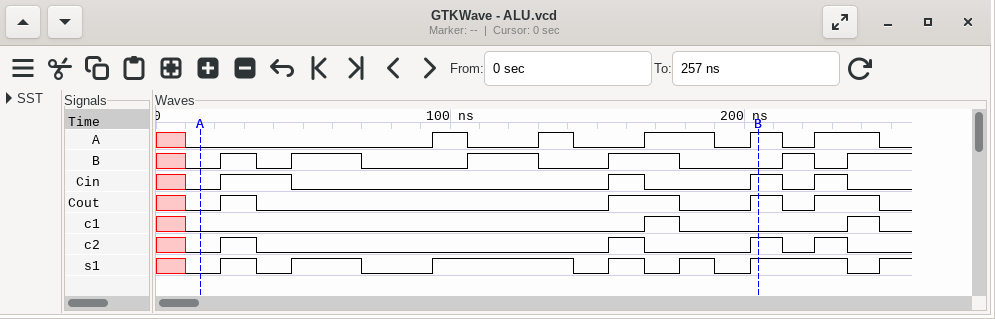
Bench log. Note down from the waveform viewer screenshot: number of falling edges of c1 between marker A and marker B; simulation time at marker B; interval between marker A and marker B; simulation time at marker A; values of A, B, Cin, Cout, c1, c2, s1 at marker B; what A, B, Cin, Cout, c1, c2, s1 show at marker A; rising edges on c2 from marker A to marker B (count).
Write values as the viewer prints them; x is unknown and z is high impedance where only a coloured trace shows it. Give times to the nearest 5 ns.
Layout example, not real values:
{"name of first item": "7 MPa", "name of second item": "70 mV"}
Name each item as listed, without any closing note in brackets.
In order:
{"number of falling edges of c1 between marker A and marker B": "1", "simulation time at marker B": "205 ns", "interval between marker A and marker B": "190 ns", "simulation time at marker A": "15 ns", "values of A, B, Cin, Cout, c1, c2, s1 at marker B": "A=1, B=0, Cin=1, Cout=1, c1=0, c2=1, s1=1", "what A, B, Cin, Cout, c1, c2, s1 show at marker A": "A=0, B=0, Cin=0, Cout=0, c1=0, c2=0, s1=0", "rising edges on c2 from marker A to marker B": "3"}
